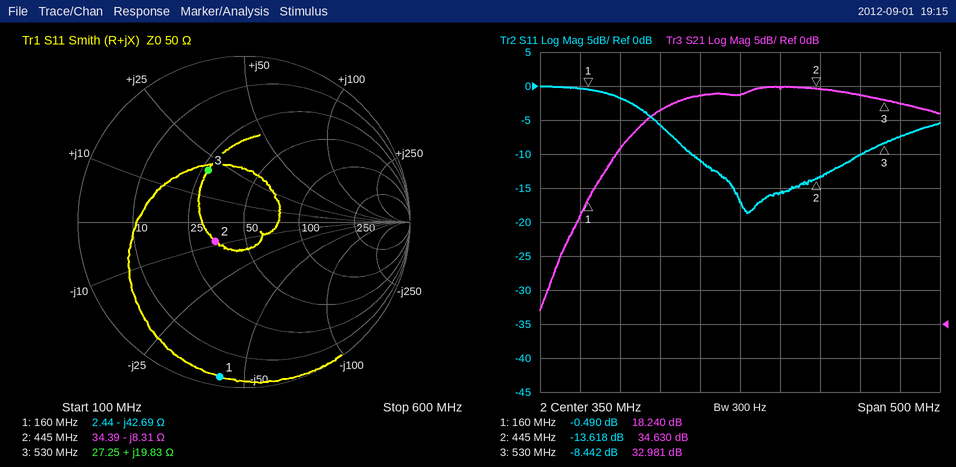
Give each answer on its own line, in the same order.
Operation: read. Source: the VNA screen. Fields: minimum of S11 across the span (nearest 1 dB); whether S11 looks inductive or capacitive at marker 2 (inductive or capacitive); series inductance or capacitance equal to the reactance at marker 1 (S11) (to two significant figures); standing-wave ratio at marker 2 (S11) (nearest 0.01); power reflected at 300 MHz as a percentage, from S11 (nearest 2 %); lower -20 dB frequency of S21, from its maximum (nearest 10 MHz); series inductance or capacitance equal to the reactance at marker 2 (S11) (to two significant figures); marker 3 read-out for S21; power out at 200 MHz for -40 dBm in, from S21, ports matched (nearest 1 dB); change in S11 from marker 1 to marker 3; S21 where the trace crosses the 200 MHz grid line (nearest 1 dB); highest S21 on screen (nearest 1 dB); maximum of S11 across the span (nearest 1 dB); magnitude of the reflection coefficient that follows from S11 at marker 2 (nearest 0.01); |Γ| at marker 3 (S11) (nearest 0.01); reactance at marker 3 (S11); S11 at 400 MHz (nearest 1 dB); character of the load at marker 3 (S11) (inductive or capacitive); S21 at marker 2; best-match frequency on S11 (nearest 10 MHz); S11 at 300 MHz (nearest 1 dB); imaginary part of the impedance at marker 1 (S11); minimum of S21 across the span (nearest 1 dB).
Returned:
-19 dB
capacitive
23 pF
1.53
8 %
150 MHz
43 pF
32.981 dB
-14 dBm
-7.952 dB
26 dB
35 dB
0 dB
0.21
0.38
+19.83 Ω
-16 dB
inductive
34.630 dB
360 MHz
-11 dB
-42.69 Ω
2 dB
